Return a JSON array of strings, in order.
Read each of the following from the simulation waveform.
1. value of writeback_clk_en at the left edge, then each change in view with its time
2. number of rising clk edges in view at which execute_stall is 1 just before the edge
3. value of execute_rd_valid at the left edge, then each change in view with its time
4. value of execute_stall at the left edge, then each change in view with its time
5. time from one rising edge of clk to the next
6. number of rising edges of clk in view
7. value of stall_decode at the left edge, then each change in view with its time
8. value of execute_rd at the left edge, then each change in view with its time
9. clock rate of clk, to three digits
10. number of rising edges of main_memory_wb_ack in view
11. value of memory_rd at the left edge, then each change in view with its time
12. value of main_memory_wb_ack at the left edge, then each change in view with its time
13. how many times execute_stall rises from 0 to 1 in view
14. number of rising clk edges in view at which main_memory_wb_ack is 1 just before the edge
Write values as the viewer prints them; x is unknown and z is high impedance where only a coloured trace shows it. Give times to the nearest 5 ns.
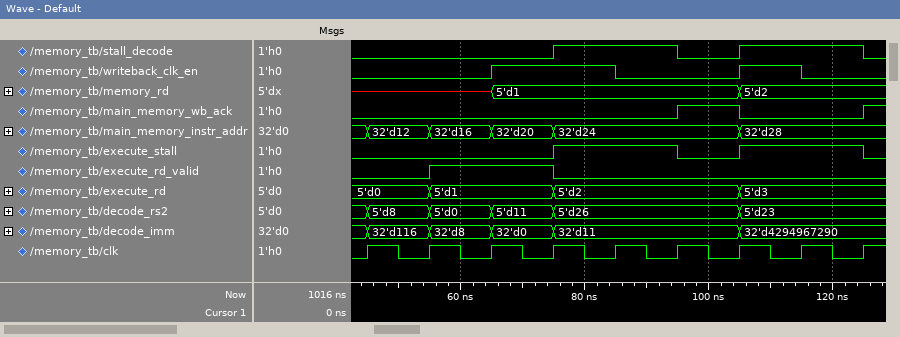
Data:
["0, 1 at 65 ns, 0 at 85 ns, 1 at 105 ns, 0 at 115 ns", "4", "0, 1 at 55 ns, 0 at 75 ns", "0, 1 at 75 ns, 0 at 95 ns, 1 at 105 ns, 0 at 125 ns", "10 ns", "9", "0, 1 at 75 ns, 0 at 95 ns, 1 at 105 ns, 0 at 125 ns", "5'd0, 5'd1 at 55 ns, 5'd2 at 75 ns, 5'd3 at 105 ns", "100 MHz", "2", "x, 5'd1 at 65 ns, 5'd2 at 105 ns", "0, 1 at 95 ns, 0 at 105 ns, 1 at 125 ns", "2", "1"]
